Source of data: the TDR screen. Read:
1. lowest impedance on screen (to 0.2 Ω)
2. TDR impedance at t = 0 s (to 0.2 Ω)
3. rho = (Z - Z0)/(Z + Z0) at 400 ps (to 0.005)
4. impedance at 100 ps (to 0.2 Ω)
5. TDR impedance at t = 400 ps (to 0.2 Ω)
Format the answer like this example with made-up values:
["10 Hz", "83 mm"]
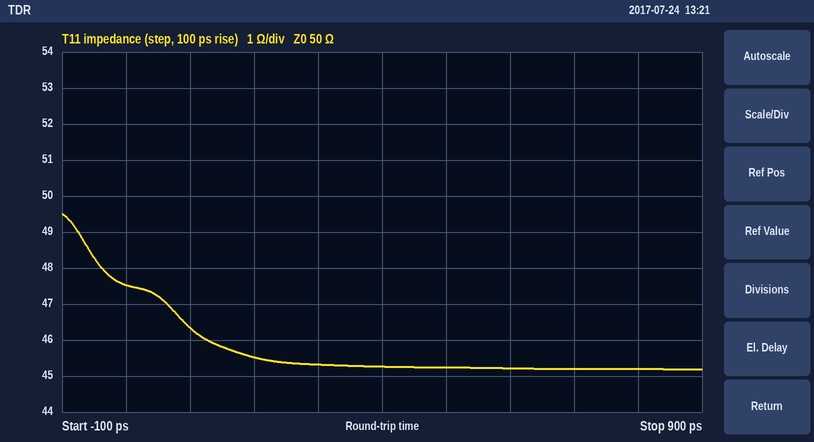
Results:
["45.2 Ω", "47.6 Ω", "-0.050", "46.4 Ω", "45.2 Ω"]
